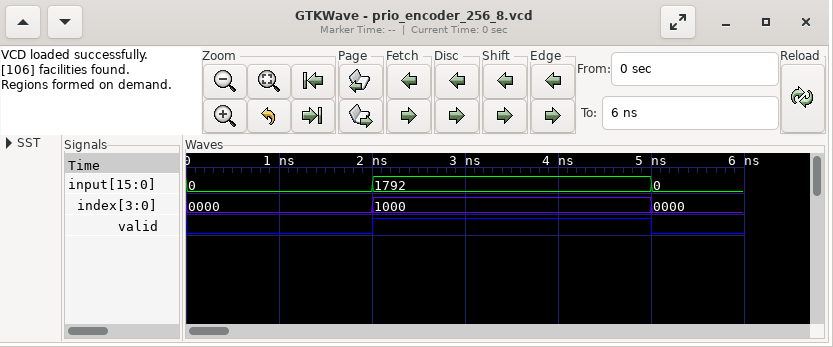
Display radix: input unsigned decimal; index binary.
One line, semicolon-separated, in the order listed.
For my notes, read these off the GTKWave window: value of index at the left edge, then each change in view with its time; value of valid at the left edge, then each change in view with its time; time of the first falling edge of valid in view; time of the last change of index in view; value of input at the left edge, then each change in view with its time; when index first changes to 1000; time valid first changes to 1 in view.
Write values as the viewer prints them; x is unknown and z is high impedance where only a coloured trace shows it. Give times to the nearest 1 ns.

0000, 1000 at 2 ns, 0000 at 5 ns; 0, 1 at 2 ns, 0 at 5 ns; 5 ns; 5 ns; 0, 1792 at 2 ns, 0 at 5 ns; 2 ns; 2 ns
